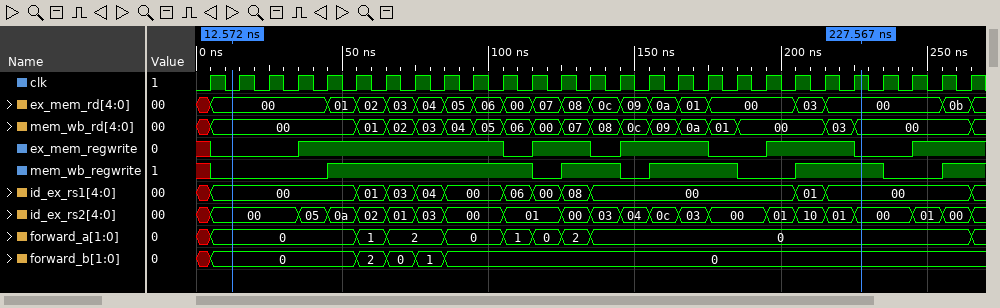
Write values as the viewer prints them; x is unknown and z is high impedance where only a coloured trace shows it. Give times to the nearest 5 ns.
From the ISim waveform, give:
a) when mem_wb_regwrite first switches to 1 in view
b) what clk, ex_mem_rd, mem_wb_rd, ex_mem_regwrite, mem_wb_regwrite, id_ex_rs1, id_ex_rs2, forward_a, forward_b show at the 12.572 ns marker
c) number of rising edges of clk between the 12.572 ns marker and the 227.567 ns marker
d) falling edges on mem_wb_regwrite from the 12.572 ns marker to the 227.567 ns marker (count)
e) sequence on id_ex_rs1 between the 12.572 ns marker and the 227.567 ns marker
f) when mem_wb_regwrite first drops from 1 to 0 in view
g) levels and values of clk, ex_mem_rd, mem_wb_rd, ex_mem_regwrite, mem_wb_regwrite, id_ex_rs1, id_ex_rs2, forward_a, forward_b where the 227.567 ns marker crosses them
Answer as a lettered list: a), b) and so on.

a) 45 ns
b) clk=0, ex_mem_rd=00, mem_wb_rd=00, ex_mem_regwrite=0, mem_wb_regwrite=0, id_ex_rs1=00, id_ex_rs2=00, forward_a=0, forward_b=0
c) 22
d) 3
e) 00, 01, 03, 04, 00, 06, 00, 08, 00, 01, 00
f) 115 ns
g) clk=1, ex_mem_rd=00, mem_wb_rd=00, ex_mem_regwrite=0, mem_wb_regwrite=1, id_ex_rs1=00, id_ex_rs2=00, forward_a=0, forward_b=0
